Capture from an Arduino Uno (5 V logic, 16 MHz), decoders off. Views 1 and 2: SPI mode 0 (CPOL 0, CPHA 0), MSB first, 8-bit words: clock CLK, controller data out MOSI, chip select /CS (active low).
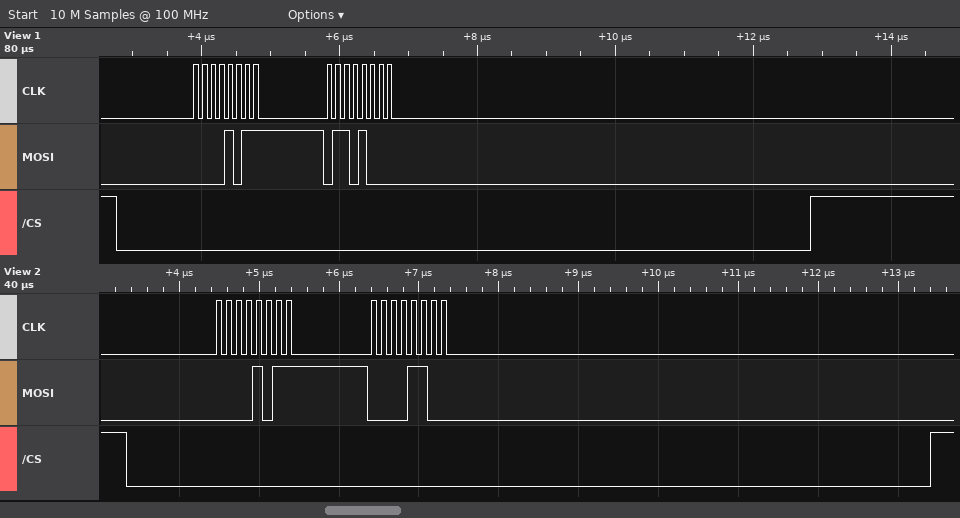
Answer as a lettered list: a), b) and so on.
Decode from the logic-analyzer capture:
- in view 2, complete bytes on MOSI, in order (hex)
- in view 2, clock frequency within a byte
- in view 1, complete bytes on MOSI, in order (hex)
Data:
a) 0B 0C
b) 8 MHz
c) 0B 68
